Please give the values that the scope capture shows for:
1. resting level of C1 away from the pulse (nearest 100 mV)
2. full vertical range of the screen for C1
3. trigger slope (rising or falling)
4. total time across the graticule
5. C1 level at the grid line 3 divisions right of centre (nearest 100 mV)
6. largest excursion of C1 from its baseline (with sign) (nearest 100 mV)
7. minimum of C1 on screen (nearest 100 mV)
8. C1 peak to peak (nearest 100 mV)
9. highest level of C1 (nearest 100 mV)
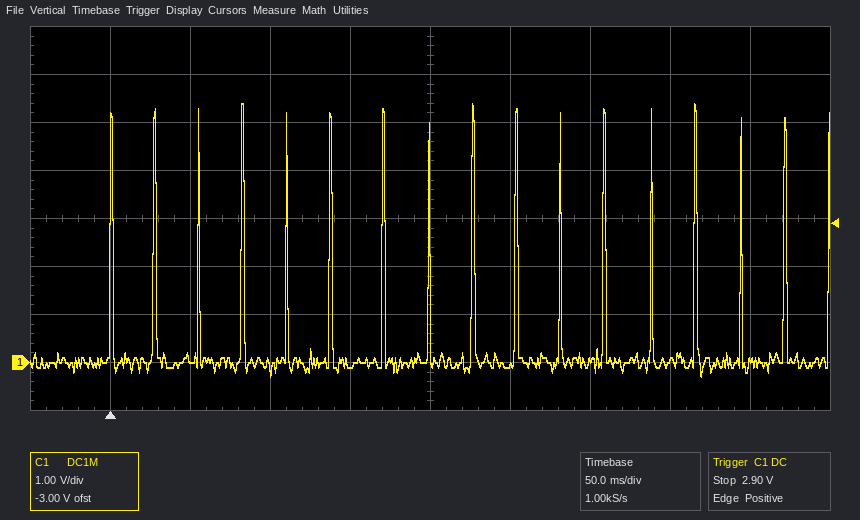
0.0 V
8 V
rising
500 ms
0.0 V
+5.4 V
-300 mV
5.7 V
5.4 V
